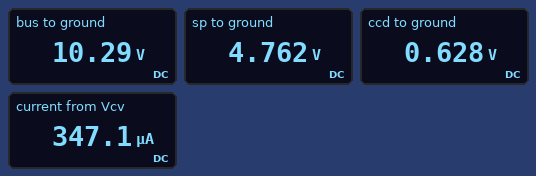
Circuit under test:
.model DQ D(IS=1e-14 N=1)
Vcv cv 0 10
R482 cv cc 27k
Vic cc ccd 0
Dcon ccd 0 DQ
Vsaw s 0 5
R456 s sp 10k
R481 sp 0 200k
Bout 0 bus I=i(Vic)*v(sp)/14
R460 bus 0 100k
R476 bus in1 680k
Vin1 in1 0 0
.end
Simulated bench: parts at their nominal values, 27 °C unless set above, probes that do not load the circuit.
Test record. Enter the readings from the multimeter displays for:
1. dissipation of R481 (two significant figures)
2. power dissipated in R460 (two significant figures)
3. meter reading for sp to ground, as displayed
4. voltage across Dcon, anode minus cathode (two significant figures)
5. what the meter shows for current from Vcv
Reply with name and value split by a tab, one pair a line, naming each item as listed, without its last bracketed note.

dissipation of R481	110 µW
power dissipated in R460	1.1 mW
meter reading for sp to ground, as displayed	4.762 V
voltage across Dcon, anode minus cathode	630 mV
what the meter shows for current from Vcv	347.1 µA
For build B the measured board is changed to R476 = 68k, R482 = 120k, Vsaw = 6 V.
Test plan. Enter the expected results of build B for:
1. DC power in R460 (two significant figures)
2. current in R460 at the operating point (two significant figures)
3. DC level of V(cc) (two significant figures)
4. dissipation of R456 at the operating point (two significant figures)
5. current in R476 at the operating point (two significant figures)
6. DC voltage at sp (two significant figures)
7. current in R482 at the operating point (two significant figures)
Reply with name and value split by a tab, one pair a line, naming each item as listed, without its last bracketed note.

DC power in R460	17 µW
current in R460 at the operating point	13 µA
DC level of V(cc)	590 mV
dissipation of R456 at the operating point	8.2 µW
current in R476 at the operating point	19 µA
DC voltage at sp	5.7 V
current in R482 at the operating point	78 µA
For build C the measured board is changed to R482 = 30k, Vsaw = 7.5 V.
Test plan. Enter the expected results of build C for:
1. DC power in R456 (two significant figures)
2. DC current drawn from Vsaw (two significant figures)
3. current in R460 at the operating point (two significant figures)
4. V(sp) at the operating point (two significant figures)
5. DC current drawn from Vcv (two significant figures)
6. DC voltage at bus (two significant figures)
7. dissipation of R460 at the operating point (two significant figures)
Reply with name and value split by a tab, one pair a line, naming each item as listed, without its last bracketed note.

DC power in R456	13 µW
DC current drawn from Vsaw	36 µA
current in R460 at the operating point	140 µA
V(sp) at the operating point	7.1 V
DC current drawn from Vcv	310 µA
DC voltage at bus	14 V
dissipation of R460 at the operating point	1.9 mW
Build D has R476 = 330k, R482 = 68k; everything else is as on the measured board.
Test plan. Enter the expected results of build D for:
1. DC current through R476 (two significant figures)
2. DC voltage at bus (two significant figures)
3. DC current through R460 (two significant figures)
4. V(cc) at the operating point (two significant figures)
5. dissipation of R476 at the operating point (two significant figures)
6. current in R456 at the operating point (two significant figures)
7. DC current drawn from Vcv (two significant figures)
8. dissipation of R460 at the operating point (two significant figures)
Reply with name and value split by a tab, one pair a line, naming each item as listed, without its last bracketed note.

DC current through R476	11 µA
DC voltage at bus	3.6 V
DC current through R460	36 µA
V(cc) at the operating point	600 mV
dissipation of R476 at the operating point	39 µW
current in R456 at the operating point	24 µA
DC current drawn from Vcv	140 µA
dissipation of R460 at the operating point	130 µW
